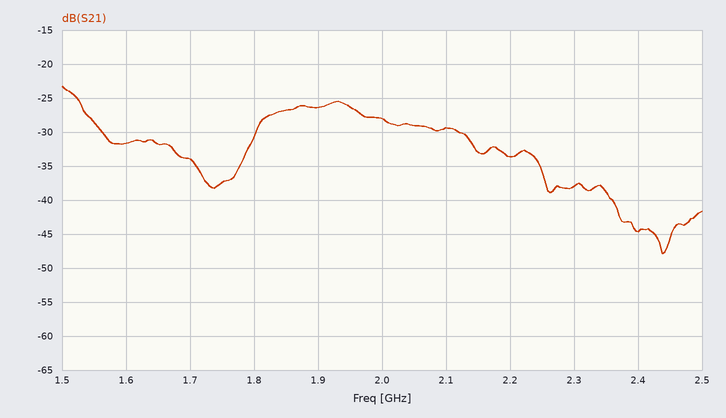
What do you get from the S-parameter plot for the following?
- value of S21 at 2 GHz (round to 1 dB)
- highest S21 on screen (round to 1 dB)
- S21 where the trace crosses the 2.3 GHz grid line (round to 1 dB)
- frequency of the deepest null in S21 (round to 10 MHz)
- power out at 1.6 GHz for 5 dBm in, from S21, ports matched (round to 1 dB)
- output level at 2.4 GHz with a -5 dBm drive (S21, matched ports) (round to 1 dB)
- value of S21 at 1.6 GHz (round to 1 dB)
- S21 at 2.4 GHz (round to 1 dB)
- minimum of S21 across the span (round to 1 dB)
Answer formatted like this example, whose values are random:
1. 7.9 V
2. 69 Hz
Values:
1. -28 dB
2. -23 dB
3. -38 dB
4. 2.44 GHz
5. -27 dBm
6. -50 dBm
7. -32 dB
8. -45 dB
9. -48 dB
